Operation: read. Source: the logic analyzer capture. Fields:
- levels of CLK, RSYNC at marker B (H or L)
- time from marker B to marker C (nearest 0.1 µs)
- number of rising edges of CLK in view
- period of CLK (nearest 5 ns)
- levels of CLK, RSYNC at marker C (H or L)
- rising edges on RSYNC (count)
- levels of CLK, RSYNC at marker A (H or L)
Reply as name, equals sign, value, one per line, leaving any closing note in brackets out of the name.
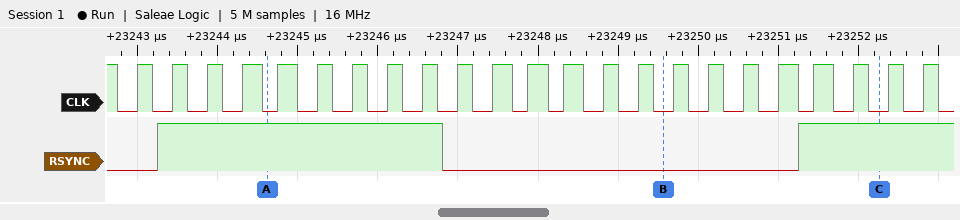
levels of CLK, RSYNC at marker B = CLK=L, RSYNC=L
time from marker B to marker C = 2.7 µs
number of rising edges of CLK in view = 23
period of CLK = 445 ns
levels of CLK, RSYNC at marker C = CLK=L, RSYNC=H
rising edges on RSYNC = 2
levels of CLK, RSYNC at marker A = CLK=L, RSYNC=H
